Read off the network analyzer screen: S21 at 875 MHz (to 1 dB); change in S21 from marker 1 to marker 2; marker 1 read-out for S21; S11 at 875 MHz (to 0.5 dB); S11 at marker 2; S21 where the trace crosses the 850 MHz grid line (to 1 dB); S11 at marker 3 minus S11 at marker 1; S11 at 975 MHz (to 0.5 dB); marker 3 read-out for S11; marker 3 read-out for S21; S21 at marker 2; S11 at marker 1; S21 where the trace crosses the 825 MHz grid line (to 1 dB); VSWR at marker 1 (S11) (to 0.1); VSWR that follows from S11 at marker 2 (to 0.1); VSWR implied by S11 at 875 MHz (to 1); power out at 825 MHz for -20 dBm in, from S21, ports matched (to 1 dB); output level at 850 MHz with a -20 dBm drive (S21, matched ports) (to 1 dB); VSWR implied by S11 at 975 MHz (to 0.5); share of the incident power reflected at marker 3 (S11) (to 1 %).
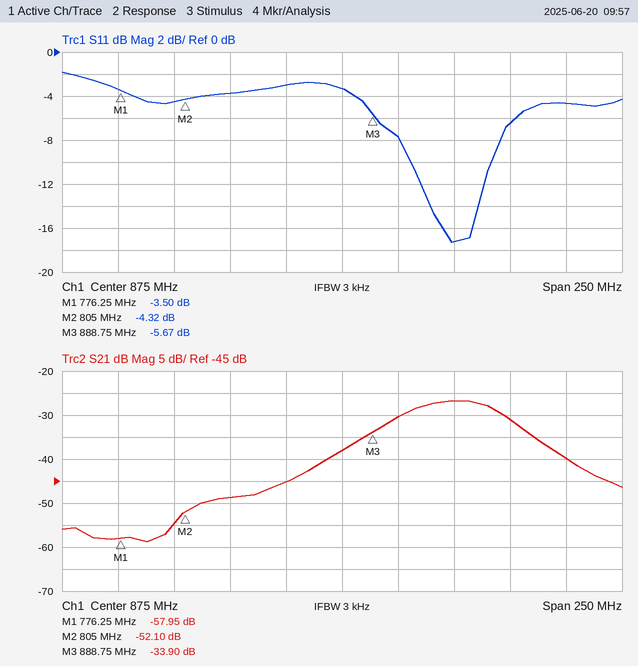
-38 dB
5.85 dB
-57.95 dB
-3.5 dB
-4.32 dB
-45 dB
-2.17 dB
-4.5 dB
-5.67 dB
-33.90 dB
-52.10 dB
-3.50 dB
-49 dB
5.0
4.1
5
-69 dBm
-65 dBm
4.0
27 %
